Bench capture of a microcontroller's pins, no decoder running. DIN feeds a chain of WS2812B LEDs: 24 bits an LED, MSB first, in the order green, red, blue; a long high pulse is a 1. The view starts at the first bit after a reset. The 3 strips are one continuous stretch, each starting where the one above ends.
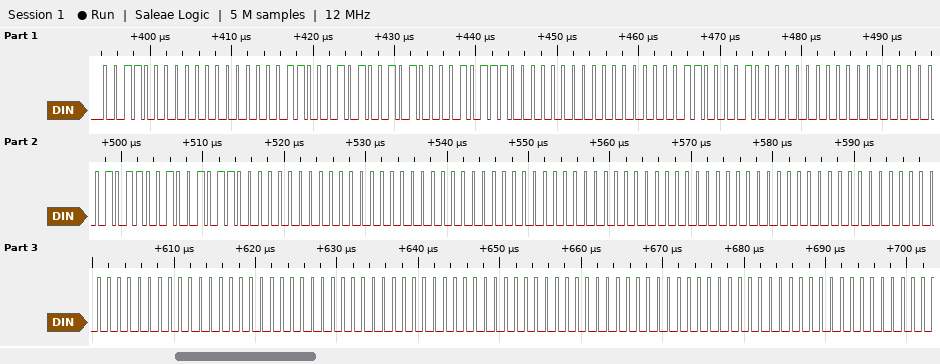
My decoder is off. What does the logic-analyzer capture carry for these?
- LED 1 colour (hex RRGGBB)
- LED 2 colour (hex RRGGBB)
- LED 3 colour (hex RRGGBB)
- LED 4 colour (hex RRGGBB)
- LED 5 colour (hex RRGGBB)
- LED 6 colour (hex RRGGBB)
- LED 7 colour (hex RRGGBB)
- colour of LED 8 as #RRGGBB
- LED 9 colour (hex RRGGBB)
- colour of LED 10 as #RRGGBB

#003031
#174A00
#610000
#16004B
#000000
#000000
#000000
#000000
#000000
#000000
